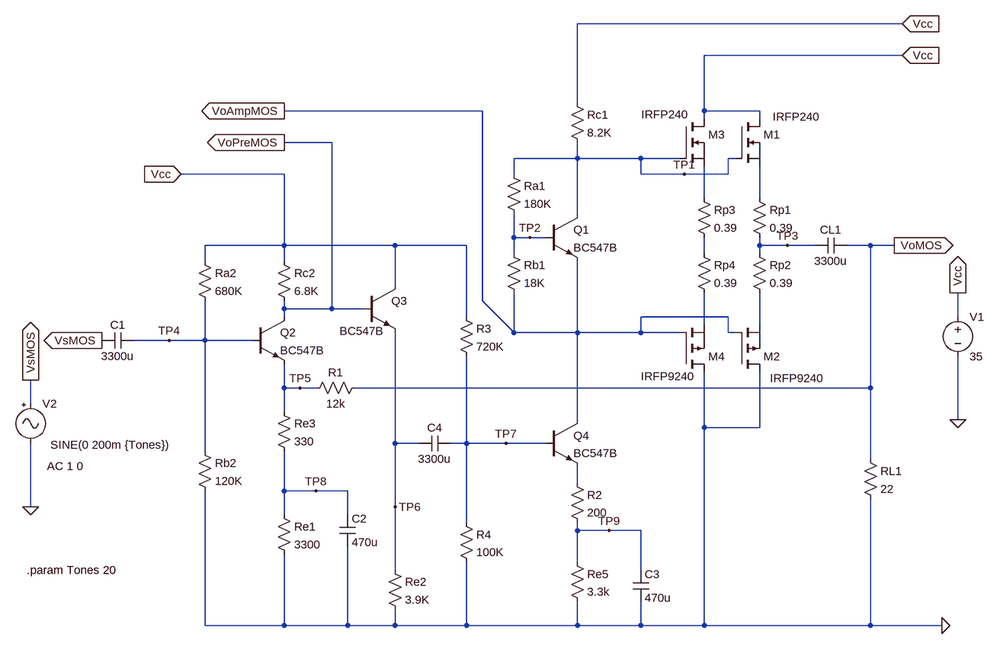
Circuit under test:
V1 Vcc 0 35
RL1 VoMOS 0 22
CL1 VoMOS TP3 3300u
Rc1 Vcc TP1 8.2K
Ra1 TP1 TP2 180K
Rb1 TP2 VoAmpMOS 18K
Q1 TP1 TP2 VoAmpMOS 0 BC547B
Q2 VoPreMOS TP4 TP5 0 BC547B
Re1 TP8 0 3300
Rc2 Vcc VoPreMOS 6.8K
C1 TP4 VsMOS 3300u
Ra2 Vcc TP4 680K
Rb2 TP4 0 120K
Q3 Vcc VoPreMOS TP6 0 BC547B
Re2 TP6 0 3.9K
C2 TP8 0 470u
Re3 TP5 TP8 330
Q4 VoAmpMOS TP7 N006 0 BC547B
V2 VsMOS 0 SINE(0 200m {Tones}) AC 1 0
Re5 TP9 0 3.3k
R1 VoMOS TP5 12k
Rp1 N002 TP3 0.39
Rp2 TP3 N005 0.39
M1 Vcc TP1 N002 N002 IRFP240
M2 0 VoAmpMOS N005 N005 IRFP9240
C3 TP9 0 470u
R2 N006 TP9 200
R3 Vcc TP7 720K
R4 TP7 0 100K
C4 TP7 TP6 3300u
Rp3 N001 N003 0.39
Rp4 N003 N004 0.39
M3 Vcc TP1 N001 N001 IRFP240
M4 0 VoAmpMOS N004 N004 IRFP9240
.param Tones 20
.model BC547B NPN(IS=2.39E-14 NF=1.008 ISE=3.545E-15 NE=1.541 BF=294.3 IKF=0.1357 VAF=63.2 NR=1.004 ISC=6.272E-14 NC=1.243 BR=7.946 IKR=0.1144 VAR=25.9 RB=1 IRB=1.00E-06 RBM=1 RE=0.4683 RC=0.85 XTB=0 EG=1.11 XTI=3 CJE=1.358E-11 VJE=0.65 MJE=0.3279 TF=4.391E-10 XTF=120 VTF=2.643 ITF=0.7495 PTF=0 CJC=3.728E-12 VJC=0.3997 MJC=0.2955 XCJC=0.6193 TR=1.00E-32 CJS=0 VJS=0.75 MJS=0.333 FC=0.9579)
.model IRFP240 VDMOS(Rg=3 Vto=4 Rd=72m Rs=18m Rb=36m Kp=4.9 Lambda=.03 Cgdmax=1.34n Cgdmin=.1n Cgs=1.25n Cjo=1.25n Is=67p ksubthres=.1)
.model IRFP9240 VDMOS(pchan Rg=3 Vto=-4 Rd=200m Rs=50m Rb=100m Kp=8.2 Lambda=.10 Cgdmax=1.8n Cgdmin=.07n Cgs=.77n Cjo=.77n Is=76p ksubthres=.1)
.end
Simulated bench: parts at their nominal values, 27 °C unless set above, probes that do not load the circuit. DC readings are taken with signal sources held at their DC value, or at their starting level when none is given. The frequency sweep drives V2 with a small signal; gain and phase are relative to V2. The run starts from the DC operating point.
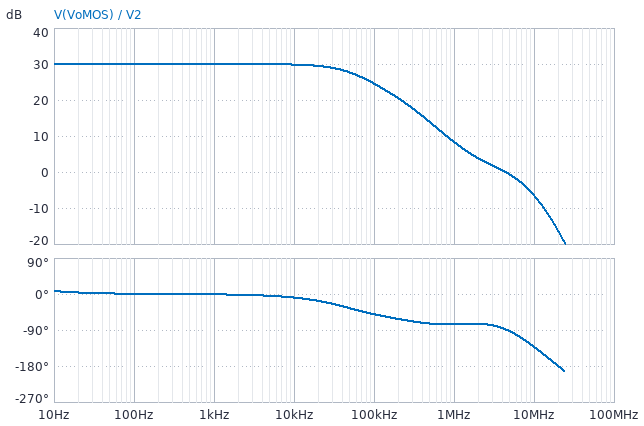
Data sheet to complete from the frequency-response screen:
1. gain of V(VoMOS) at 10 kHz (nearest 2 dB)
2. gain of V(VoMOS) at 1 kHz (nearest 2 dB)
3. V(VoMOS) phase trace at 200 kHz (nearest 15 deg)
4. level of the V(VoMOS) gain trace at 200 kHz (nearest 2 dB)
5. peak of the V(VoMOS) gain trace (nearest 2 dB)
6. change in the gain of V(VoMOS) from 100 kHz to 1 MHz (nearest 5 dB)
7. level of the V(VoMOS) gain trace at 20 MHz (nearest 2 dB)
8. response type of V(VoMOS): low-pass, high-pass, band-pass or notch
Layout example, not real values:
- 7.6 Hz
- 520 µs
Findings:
- 30 dB
- 30 dB
- -60 deg
- 20 dB
- 30 dB
- -15 dB
- -16 dB
- low-pass
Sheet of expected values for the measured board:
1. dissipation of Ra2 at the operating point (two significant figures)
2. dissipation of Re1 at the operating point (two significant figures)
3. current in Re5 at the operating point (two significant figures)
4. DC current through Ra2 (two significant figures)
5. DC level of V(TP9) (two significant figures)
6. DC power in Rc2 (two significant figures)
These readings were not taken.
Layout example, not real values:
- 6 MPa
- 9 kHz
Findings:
- 1.3 mW
- 4.4 mW
- 970 µA
- 44 µA
- 3.2 V
- 16 mW
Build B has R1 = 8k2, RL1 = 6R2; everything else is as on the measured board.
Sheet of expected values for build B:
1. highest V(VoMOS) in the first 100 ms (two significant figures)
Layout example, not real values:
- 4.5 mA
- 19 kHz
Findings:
- 4.7 V
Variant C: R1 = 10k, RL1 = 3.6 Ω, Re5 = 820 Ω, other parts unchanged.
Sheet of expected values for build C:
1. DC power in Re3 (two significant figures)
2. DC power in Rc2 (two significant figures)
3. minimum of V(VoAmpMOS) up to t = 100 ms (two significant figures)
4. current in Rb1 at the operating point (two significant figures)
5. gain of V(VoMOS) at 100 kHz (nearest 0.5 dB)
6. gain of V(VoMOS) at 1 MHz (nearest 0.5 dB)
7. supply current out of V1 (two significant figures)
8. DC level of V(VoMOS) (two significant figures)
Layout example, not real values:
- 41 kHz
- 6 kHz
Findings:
- 440 µW
- 17 mW
- 2.8 V
- 37 µA
- 29.5 dB
- 24.0 dB
- 730 mA
- 1.5 mV
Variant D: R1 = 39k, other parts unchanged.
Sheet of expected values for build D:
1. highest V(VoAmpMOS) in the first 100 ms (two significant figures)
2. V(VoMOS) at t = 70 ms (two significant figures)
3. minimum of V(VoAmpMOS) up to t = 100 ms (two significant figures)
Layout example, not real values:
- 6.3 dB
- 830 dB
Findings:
- 35 V
- 7.1 V
- 3.8 V
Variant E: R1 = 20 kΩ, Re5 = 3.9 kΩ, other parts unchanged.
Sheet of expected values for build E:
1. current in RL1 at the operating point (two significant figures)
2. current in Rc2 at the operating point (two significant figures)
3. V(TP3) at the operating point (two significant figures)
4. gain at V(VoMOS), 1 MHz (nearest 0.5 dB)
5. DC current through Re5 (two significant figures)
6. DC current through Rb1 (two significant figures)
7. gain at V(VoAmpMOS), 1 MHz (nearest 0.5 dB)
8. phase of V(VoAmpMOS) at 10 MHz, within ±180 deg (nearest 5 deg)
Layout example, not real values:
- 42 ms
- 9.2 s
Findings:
- 210 µA
- 1.4 mA
- 24 V
- 3.0 dB
- 840 µA
- 35 µA
- 20.0 dB
- -140 deg
